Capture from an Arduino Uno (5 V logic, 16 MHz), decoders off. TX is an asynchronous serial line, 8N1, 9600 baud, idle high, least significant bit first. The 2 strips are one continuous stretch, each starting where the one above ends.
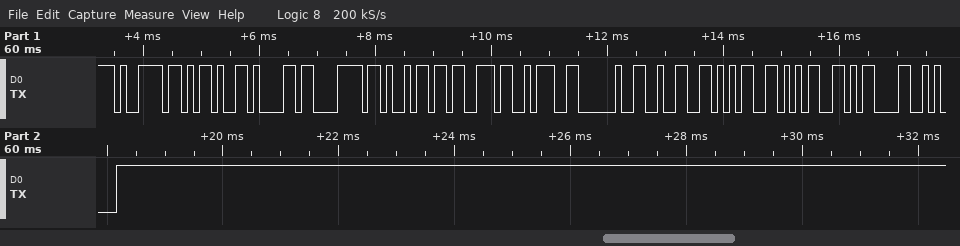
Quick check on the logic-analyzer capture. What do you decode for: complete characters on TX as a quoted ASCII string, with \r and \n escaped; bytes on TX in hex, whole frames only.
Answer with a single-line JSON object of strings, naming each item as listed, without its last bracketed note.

{"complete characters on TX as a quoted ASCII string, with \\r and \\n escaped": "\"y-axis: 255\\r\\n\"", "bytes on TX in hex, whole frames only": "79 2D 61 78 69 73 3A 20 32 35 35 0D 0A"}
